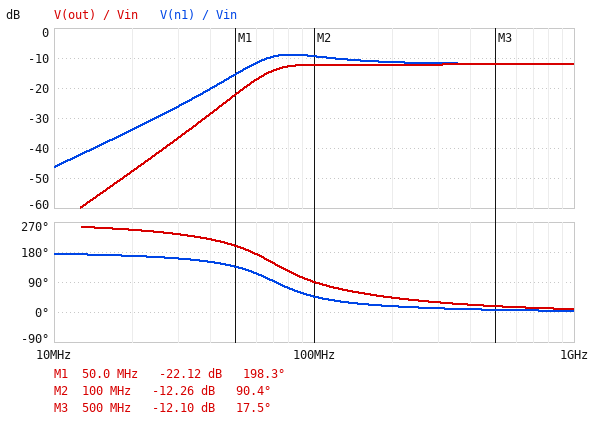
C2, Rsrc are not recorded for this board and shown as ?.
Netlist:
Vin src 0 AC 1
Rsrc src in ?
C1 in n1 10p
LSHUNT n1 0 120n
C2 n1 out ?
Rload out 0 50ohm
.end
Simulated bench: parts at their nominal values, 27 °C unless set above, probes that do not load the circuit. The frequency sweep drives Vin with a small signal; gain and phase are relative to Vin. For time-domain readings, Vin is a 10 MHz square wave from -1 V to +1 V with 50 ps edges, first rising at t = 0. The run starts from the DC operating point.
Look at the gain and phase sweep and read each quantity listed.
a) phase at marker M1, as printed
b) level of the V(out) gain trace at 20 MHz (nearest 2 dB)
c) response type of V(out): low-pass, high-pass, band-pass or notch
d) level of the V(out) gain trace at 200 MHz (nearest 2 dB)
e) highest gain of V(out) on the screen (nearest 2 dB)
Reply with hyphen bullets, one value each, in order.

- 198.3 deg
- -48 dB
- high-pass
- -12 dB
- -12 dB
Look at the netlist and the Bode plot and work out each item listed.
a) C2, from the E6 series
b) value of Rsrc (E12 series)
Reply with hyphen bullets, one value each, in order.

- 33 pF
- 150 Ω
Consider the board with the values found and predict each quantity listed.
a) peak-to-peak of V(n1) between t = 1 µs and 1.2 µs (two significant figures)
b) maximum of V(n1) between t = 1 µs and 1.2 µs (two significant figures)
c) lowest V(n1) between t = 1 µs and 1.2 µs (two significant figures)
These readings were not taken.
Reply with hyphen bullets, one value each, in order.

- 990 mV
- 500 mV
- -500 mV
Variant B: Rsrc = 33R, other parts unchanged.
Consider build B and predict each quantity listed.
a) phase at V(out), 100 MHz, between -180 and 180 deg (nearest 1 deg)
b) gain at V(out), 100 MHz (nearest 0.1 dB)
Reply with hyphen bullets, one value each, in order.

- 109 deg
- -8.6 dB
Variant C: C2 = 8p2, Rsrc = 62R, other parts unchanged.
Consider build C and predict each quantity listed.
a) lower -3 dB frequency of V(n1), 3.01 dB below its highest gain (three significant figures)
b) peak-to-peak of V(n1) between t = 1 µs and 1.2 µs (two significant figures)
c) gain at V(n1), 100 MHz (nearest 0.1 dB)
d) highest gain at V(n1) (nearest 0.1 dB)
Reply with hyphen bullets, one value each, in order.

- 95.1 MHz
- 1.8 V
- 2.3 dB
- 3.8 dB
